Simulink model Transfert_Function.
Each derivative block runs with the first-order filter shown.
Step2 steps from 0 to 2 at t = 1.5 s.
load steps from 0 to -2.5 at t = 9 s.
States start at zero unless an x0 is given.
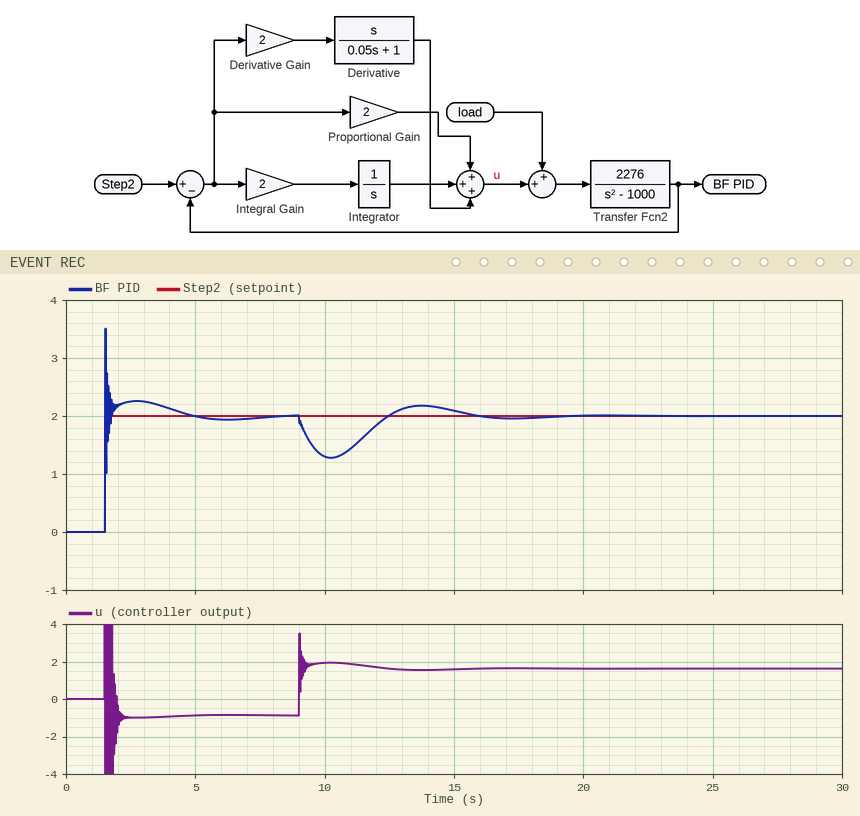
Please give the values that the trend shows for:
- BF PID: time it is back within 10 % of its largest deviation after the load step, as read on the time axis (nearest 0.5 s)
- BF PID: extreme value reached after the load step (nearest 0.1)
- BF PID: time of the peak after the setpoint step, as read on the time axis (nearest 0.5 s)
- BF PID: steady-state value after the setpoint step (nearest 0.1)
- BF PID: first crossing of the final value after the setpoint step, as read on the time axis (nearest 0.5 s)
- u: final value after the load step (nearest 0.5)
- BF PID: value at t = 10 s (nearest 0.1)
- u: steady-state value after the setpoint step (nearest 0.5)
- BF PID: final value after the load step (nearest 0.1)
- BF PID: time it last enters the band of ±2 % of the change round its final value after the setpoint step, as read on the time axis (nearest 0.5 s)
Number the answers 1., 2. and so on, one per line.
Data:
1. 15.0 s
2. 1.3
3. 1.5 s
4. 2.0
5. 1.5 s
6. 1.5
7. 1.3
8. -1.0
9. 2.0
10. 7.5 s
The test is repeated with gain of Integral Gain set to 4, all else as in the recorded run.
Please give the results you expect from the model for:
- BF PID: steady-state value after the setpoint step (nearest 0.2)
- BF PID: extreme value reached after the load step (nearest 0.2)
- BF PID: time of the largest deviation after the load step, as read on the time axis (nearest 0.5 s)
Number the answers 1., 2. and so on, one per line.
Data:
1. 2.0
2. 1.4
3. 10.0 s
